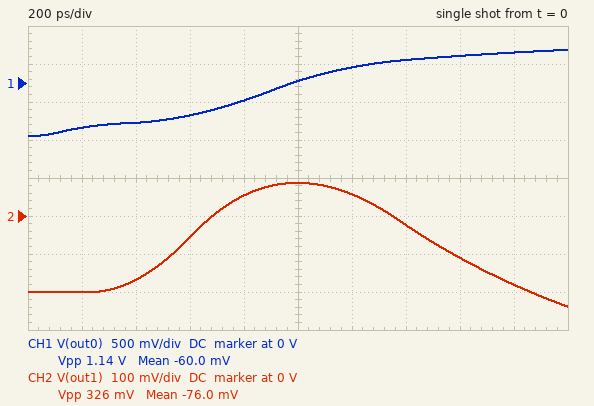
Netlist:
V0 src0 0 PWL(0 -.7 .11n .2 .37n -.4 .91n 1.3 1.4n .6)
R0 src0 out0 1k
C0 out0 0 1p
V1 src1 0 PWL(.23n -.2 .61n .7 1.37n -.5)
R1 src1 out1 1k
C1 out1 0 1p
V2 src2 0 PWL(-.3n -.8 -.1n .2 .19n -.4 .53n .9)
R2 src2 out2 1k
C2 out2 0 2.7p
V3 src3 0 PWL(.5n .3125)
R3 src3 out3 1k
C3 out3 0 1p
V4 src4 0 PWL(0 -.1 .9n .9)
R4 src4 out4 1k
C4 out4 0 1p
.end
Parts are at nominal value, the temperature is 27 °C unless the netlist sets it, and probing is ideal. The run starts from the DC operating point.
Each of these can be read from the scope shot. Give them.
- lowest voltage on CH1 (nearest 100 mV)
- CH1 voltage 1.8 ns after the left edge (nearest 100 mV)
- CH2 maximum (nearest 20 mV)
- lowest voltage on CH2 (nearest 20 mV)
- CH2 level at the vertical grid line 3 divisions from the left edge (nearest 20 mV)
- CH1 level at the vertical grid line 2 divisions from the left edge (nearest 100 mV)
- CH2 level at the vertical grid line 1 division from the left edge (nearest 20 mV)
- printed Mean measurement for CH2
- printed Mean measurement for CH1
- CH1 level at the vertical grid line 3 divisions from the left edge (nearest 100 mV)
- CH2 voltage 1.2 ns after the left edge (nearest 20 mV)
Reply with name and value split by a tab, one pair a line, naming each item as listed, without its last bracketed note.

lowest voltage on CH1	-700 mV
CH1 voltage 1.8 ns after the left edge	400 mV
CH2 maximum	80 mV
lowest voltage on CH2	-240 mV
CH2 level at the vertical grid line 3 divisions from the left edge	-60 mV
CH1 level at the vertical grid line 2 divisions from the left edge	-500 mV
CH2 level at the vertical grid line 1 division from the left edge	-200 mV
printed Mean measurement for CH2	-76.0 mV
printed Mean measurement for CH1	-60.0 mV
CH1 level at the vertical grid line 3 divisions from the left edge	-400 mV
CH2 voltage 1.2 ns after the left edge	60 mV
